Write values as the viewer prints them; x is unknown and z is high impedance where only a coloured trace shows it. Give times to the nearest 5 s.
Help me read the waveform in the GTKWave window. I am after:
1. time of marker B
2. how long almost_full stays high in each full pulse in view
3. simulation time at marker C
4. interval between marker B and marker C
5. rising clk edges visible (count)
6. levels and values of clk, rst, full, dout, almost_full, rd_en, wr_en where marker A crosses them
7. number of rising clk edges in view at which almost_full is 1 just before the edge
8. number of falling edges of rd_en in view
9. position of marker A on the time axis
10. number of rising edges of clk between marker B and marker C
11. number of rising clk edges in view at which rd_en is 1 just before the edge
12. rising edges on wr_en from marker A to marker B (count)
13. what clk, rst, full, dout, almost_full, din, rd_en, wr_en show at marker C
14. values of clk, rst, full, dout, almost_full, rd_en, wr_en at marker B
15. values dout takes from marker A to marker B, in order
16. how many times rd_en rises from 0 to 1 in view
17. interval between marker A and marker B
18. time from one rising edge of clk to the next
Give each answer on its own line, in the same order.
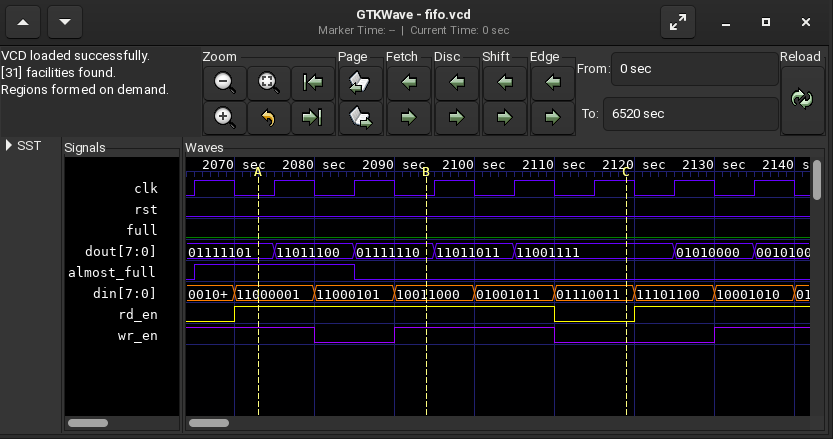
2095 s
20 s
2120 s
25 s
8
clk=0, rst=0, full=0, dout=01111101, almost_full=1, rd_en=1, wr_en=1
2
1
2075 s
3
6
1
clk=1, rst=0, full=0, dout=11001111, almost_full=0, din=01110011, rd_en=0, wr_en=0
clk=0, rst=0, full=0, dout=01111110, almost_full=0, rd_en=1, wr_en=1
01111101, 11011100, 01111110
2
20 s
10 s
